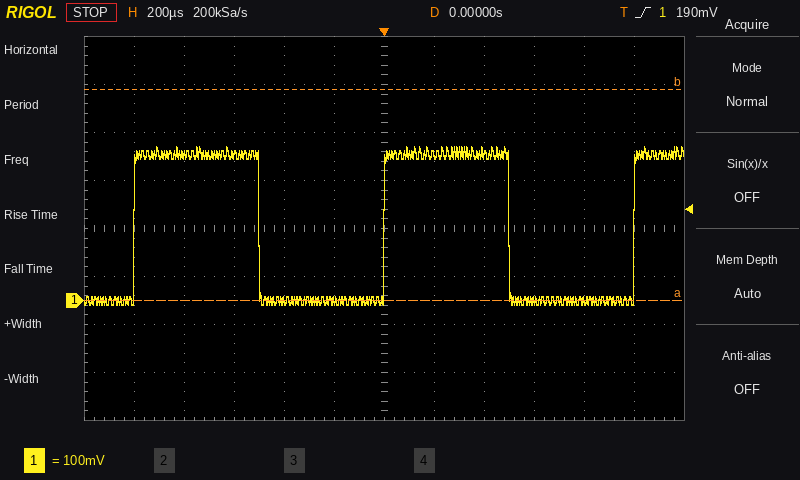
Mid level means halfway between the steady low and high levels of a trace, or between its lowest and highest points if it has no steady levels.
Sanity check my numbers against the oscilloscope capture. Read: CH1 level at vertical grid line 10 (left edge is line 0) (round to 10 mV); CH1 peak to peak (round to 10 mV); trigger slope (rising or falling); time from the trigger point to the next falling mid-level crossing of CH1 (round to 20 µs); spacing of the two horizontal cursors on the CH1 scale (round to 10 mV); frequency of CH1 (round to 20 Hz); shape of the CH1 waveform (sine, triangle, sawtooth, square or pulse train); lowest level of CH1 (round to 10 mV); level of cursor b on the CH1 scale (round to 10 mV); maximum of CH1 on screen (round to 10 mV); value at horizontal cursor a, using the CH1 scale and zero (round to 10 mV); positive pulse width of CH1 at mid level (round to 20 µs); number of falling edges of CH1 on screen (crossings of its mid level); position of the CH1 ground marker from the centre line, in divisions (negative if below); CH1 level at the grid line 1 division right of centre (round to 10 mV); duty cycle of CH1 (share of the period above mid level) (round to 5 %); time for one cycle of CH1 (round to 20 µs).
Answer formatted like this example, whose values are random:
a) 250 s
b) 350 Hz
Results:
a) 0 mV
b) 330 mV
c) rising
d) 500 µs
e) 440 mV
f) 1.00 kHz
g) square
h) -10 mV
i) 440 mV
j) 320 mV
k) 0 mV
l) 500 µs
m) 2
n) -1.5 div
o) 300 mV
p) 50 %
q) 1.00 ms
